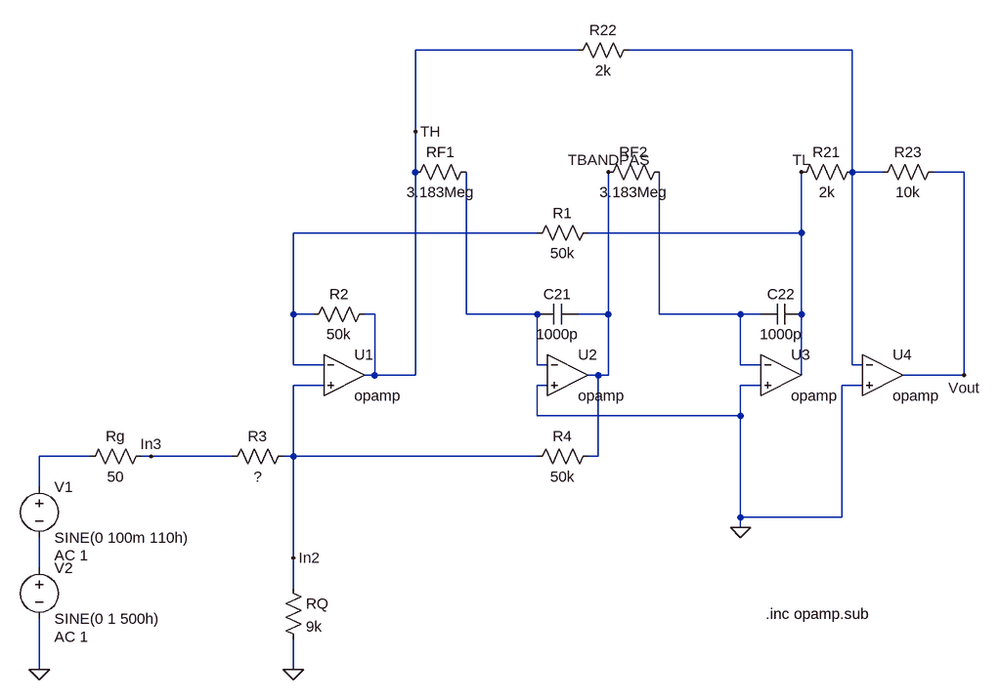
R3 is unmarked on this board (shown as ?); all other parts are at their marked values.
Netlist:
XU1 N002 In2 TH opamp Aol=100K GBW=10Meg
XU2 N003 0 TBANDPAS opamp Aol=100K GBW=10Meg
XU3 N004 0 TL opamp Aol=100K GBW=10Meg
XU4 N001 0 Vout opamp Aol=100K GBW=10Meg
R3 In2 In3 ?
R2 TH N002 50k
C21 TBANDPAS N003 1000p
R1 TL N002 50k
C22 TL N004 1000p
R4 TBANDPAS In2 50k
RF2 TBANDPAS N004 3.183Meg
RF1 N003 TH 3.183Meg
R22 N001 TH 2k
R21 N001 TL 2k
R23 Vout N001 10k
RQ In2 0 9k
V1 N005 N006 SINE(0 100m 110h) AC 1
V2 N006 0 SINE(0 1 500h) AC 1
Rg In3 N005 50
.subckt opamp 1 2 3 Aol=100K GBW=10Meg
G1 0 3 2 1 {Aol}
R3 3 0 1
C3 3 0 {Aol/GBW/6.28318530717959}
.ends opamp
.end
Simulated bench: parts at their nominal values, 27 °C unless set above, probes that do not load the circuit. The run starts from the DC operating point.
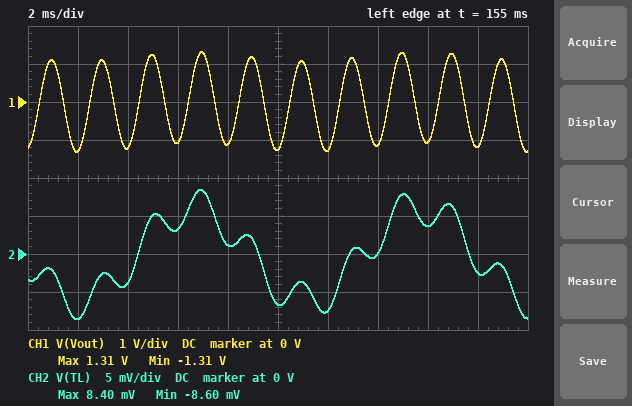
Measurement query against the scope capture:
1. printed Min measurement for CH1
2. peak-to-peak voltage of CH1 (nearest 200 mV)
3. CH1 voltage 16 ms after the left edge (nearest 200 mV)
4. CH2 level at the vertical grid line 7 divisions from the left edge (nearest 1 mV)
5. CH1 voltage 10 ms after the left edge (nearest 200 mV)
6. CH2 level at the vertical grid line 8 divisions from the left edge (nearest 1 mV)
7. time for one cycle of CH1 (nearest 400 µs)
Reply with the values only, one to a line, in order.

-1.31 V
2.6 V
-1.0 V
0 V
-1.2 V
4 mV
2.0 ms
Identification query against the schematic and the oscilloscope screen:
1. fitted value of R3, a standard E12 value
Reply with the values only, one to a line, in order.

56 kΩ
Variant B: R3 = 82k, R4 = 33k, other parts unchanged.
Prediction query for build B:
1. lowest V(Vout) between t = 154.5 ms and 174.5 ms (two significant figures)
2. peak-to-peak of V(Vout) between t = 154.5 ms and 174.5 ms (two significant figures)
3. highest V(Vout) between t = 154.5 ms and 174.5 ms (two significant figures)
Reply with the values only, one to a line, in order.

-870 mV
1.7 V
870 mV
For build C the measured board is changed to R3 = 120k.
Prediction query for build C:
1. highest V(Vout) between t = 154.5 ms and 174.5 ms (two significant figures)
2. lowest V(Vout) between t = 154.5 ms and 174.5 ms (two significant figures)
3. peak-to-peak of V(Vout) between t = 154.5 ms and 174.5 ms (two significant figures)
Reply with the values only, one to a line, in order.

650 mV
-660 mV
1.3 V
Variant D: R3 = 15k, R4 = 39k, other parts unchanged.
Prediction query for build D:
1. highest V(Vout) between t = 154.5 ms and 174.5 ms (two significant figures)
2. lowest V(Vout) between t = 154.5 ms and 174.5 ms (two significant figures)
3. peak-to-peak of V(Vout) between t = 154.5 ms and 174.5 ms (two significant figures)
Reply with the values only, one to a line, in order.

3.6 V
-3.6 V
7.2 V
